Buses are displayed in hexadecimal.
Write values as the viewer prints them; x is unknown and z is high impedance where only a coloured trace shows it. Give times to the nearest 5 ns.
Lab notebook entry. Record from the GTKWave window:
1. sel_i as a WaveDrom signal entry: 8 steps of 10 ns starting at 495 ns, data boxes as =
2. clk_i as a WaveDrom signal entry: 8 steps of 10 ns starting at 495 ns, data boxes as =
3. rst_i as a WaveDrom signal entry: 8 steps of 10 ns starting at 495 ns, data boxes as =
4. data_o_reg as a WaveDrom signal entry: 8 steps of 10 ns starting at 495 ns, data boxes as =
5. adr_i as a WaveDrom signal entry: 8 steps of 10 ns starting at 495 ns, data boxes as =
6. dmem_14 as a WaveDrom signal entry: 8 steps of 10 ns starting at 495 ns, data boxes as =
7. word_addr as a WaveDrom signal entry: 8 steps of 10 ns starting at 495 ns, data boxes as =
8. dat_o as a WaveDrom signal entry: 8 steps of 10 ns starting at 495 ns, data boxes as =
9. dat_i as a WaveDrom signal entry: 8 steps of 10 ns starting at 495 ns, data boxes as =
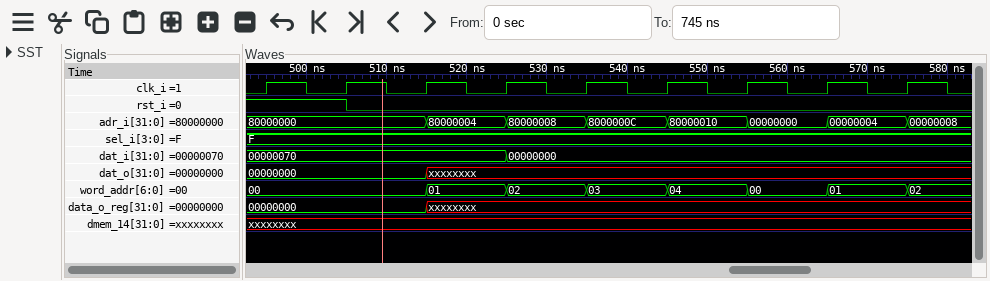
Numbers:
{name: 'sel_i', wave: '=.......', data: 'F'}
{name: 'clk_i', wave: 'p.......'}
{name: 'rst_i', wave: '10......'}
{name: 'data_o_reg', wave: '=.x.....', data: '00000000'}
{name: 'adr_i', wave: '=.======', data: '80000000 80000004 80000008 8000000C 80000010 00000000 00000004'}
{name: 'dmem_14', wave: 'x.......'}
{name: 'word_addr', wave: '=.======', data: '00 01 02 03 04 00 01'}
{name: 'dat_o', wave: '=.x.....', data: '00000000'}
{name: 'dat_i', wave: '=..=....', data: '00000070 00000000'}
